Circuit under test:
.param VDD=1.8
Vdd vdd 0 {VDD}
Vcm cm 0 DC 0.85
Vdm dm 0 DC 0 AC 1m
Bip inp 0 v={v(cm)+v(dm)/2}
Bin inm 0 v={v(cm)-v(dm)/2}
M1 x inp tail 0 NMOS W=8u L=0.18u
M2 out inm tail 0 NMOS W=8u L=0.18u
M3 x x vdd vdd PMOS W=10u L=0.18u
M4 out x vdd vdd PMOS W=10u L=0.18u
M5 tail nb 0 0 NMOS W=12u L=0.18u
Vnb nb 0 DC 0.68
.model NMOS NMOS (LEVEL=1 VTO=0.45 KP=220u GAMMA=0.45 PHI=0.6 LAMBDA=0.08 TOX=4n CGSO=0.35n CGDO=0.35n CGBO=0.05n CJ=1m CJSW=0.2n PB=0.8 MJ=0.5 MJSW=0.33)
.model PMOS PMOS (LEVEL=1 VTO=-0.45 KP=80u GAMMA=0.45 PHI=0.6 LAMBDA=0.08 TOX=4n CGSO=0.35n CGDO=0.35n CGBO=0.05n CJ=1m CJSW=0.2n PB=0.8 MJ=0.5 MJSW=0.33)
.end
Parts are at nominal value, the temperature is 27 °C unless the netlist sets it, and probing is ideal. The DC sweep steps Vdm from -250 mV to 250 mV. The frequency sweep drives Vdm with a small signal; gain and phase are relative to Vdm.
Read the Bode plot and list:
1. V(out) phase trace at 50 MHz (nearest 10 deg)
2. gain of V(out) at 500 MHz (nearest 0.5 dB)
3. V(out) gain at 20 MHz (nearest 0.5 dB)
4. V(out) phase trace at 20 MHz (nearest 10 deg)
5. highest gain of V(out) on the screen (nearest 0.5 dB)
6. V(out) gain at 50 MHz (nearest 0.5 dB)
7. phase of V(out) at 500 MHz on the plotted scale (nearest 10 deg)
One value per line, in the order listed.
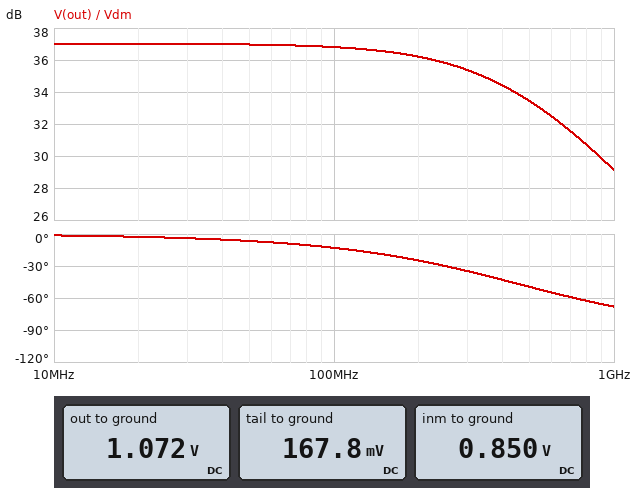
-10 deg
33.5 dB
37.0 dB
0 deg
37.0 dB
37.0 dB
-50 deg
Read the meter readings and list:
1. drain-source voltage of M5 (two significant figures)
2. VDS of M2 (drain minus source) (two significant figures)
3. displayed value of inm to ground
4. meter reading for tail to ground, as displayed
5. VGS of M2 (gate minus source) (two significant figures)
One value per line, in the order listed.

170 mV
900 mV
0.850 V
167.8 mV
680 mV
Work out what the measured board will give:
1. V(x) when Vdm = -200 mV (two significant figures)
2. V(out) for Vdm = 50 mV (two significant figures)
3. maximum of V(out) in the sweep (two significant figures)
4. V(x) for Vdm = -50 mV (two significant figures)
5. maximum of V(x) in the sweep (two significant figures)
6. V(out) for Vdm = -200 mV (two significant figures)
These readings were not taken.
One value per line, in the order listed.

1.1 V
1.7 V
1.8 V
1.1 V
1.1 V
150 mV
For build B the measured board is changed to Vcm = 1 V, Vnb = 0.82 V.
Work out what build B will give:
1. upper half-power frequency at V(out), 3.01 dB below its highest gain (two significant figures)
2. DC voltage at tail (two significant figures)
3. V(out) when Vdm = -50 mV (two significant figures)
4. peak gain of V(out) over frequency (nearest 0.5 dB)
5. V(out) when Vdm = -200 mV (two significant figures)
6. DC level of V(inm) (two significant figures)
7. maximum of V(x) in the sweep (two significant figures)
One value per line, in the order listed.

1.0 GHz
210 mV
370 mV
33.5 dB
240 mV
1.0 V
990 mV
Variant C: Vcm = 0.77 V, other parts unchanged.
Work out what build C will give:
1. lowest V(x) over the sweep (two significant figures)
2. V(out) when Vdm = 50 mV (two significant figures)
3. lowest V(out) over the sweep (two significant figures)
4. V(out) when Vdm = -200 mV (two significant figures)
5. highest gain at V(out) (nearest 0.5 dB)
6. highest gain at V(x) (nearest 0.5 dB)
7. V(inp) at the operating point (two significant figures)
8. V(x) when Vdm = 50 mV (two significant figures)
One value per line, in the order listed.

970 mV
1.7 V
81 mV
100 mV
38.0 dB
-6.5 dB
770 mV
1.1 V
